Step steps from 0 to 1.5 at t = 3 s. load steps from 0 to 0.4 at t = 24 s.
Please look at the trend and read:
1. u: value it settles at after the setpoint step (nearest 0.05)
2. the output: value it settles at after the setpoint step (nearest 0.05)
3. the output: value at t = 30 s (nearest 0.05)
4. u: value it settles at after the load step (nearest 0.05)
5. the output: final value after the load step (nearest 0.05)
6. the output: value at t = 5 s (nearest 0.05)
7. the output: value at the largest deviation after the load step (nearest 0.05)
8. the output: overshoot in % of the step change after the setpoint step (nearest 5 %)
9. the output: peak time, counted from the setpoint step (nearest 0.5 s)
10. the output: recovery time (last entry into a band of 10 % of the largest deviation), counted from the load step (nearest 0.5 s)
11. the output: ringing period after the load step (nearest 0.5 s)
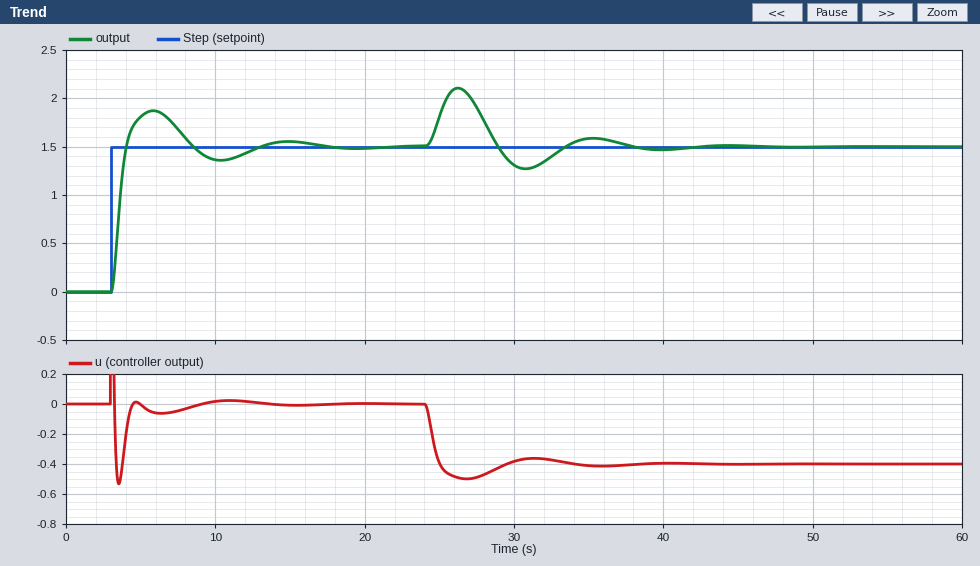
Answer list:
0.00
1.50
1.30
-0.40
1.50
1.80
2.10
25 %
3.0 s
12.5 s
9.0 s
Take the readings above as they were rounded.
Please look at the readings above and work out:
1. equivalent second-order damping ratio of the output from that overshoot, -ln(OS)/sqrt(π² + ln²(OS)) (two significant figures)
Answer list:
0.40
